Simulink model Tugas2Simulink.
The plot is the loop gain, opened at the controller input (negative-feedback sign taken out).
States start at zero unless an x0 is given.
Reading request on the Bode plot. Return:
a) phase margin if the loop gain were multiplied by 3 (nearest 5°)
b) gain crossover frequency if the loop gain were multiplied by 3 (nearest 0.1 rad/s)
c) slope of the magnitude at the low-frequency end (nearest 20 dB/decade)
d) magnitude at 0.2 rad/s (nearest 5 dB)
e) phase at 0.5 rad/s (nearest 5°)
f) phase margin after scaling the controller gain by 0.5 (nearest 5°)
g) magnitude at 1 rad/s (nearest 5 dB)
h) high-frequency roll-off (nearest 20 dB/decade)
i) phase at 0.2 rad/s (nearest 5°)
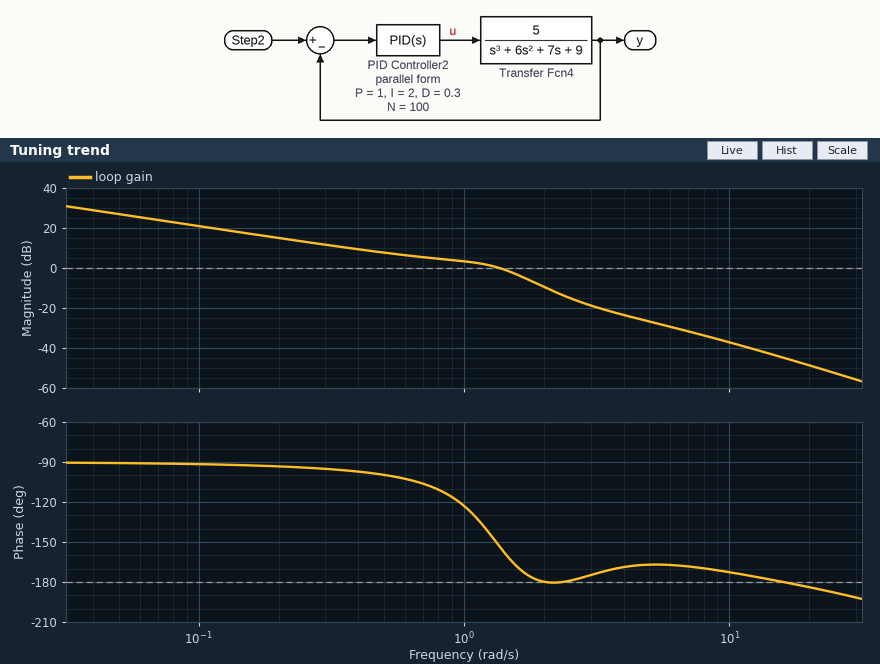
0°
2.0 rad/s
-20 dB/decade
15 dB
-100°
75°
5 dB
-40 dB/decade
-95°
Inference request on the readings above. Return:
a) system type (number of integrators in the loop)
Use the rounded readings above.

1
